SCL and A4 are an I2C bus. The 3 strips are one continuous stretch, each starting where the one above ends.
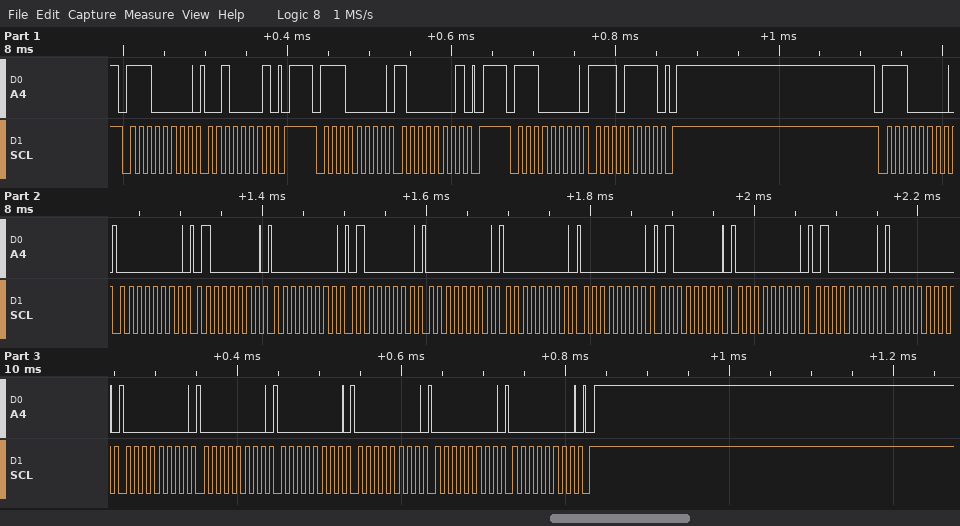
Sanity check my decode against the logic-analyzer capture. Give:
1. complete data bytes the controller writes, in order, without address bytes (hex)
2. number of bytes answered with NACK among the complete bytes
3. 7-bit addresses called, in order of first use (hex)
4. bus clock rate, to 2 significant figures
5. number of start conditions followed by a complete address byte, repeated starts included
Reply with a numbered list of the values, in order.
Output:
1. 21 81 EF 00 40 00 40 00 00 00 40 00 40 00 00 00 00 00 00 00
2. 0
3. 0x70
4. 100 kHz
5. 4
